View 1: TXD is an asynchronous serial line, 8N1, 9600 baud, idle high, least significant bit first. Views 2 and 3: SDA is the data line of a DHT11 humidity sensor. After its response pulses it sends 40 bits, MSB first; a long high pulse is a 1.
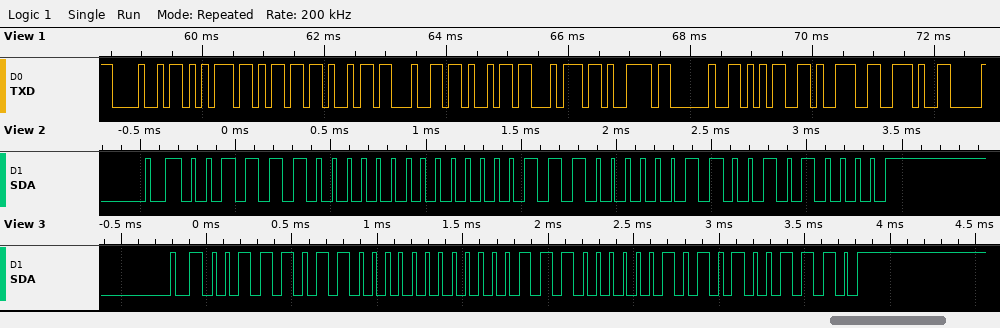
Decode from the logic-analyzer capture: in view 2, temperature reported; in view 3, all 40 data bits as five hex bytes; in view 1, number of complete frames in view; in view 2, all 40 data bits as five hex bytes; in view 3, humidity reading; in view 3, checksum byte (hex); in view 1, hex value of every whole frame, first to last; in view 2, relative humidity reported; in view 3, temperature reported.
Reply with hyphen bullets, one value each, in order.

- 14.6 °C
- 3B 00 0E 05 4E
- 12
- 3C 00 0E 06 50
- 59 %
- 0x4E
- 0x48 0x75 0x6D 0x69 0x64 0x69 0x74 0x79 0x20 0x35 0x39 0x2E
- 60 %
- 14.5 °C
